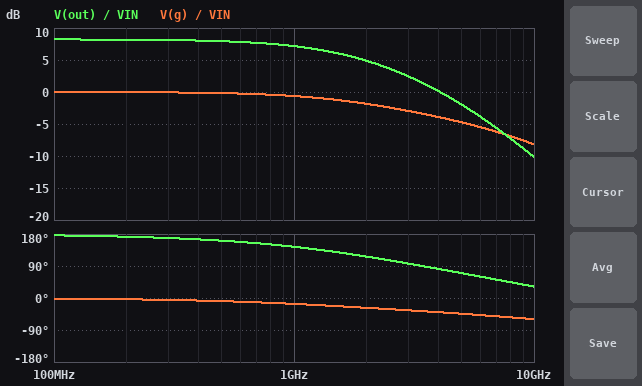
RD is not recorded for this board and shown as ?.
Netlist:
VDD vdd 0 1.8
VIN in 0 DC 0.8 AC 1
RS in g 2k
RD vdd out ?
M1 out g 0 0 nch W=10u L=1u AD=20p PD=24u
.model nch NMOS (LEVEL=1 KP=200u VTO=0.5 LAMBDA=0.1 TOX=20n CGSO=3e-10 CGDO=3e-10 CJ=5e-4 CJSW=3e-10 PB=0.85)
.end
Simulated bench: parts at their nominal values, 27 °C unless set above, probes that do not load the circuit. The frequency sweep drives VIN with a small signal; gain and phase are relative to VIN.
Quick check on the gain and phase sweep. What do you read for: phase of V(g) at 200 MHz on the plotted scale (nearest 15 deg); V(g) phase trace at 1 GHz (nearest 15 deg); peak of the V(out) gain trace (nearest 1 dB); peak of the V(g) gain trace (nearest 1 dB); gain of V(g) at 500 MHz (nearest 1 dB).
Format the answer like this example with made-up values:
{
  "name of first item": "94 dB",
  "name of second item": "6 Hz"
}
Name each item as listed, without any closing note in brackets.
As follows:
{
  "phase of V(g) at 200 MHz on the plotted scale": "0 deg",
  "V(g) phase trace at 1 GHz": "-15 deg",
  "peak of the V(out) gain trace": "8 dB",
  "peak of the V(g) gain trace": "0 dB",
  "gain of V(g) at 500 MHz": "0 dB"
}
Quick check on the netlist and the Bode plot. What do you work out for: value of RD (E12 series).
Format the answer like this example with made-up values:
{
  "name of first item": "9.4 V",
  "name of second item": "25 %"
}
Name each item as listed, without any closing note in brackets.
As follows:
{
  "value of RD": "3.9 kΩ"
}
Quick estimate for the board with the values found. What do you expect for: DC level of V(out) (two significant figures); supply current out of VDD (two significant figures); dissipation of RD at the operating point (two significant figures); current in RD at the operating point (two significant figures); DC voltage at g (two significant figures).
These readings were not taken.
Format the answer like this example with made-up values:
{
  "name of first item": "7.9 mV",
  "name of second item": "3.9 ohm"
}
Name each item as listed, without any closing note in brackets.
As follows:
{
  "DC level of V(out)": "1.4 V",
  "supply current out of VDD": "100 µA",
  "dissipation of RD at the operating point": "41 µW",
  "current in RD at the operating point": "100 µA",
  "DC voltage at g": "800 mV"
}
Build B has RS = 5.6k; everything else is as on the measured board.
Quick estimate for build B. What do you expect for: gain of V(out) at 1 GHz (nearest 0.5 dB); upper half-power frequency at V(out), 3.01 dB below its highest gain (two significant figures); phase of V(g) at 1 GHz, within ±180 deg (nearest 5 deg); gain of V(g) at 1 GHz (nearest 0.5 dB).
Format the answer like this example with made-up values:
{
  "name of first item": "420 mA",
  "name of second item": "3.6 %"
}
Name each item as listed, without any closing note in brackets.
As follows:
{
  "gain of V(out) at 1 GHz": "5.0 dB",
  "upper half-power frequency at V(out), 3.01 dB below its highest gain": "950 MHz",
  "phase of V(g) at 1 GHz, within ±180 deg": "-40 deg",
  "gain of V(g) at 1 GHz": "-3.0 dB"
}
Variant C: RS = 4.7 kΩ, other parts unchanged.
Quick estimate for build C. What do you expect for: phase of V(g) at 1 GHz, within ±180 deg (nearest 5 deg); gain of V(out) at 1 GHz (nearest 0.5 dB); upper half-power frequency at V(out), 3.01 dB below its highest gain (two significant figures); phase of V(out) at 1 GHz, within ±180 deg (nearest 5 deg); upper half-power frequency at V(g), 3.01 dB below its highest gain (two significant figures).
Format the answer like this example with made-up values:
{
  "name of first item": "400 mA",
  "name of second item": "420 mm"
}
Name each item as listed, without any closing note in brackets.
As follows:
{
  "phase of V(g) at 1 GHz, within ±180 deg": "-35 deg",
  "gain of V(out) at 1 GHz": "5.5 dB",
  "upper half-power frequency at V(out), 3.01 dB below its highest gain": "1.1 GHz",
  "phase of V(out) at 1 GHz, within ±180 deg": "125 deg",
  "upper half-power frequency at V(g), 3.01 dB below its highest gain": "1.2 GHz"
}
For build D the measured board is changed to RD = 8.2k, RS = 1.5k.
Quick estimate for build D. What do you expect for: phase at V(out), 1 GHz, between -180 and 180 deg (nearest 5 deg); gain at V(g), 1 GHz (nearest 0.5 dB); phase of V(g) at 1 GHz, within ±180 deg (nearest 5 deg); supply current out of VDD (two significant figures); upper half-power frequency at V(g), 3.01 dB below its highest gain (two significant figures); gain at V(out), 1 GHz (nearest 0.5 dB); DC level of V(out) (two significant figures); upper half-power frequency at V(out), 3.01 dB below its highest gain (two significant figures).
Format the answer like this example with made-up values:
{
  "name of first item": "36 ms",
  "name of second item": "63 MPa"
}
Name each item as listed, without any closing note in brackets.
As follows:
{
  "phase at V(out), 1 GHz, between -180 and 180 deg": "130 deg",
  "gain at V(g), 1 GHz": "-1.0 dB",
  "phase of V(g) at 1 GHz, within ±180 deg": "-15 deg",
  "supply current out of VDD": "99 µA",
  "upper half-power frequency at V(g), 3.01 dB below its highest gain": "4.4 GHz",
  "gain at V(out), 1 GHz": "11.5 dB",
  "DC level of V(out)": "990 mV",
  "upper half-power frequency at V(out), 3.01 dB below its highest gain": "1.1 GHz"
}
